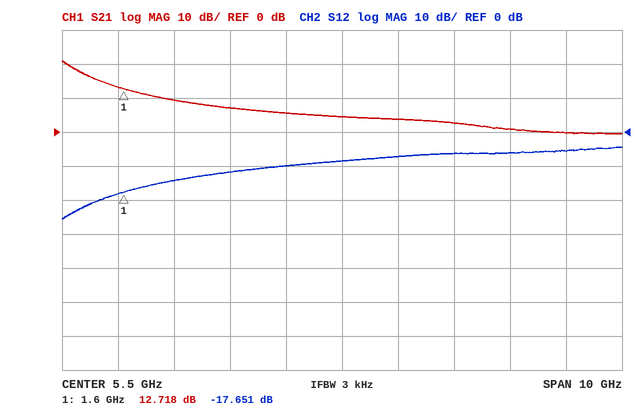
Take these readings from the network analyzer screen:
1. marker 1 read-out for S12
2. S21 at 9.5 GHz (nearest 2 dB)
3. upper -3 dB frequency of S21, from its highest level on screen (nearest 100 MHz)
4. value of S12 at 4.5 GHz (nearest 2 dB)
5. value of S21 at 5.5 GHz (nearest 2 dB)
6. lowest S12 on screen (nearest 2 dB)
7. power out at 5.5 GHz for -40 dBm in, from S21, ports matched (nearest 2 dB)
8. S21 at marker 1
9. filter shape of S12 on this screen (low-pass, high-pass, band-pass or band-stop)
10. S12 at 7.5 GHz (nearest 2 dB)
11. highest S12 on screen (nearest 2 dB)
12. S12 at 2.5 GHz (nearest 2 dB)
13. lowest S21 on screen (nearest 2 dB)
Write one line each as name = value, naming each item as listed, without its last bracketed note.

marker 1 read-out for S12 = -17.651 dB
S21 at 9.5 GHz = 0 dB
upper -3 dB frequency of S21, from its highest level on screen = 800 MHz
value of S12 at 4.5 GHz = -10 dB
value of S21 at 5.5 GHz = 4 dB
lowest S12 on screen = -26 dB
power out at 5.5 GHz for -40 dBm in, from S21, ports matched = -36 dBm
S21 at marker 1 = 12.718 dB
filter shape of S12 on this screen = high-pass
S12 at 7.5 GHz = -6 dB
highest S12 on screen = -4 dB
S12 at 2.5 GHz = -14 dB
lowest S21 on screen = 0 dB
